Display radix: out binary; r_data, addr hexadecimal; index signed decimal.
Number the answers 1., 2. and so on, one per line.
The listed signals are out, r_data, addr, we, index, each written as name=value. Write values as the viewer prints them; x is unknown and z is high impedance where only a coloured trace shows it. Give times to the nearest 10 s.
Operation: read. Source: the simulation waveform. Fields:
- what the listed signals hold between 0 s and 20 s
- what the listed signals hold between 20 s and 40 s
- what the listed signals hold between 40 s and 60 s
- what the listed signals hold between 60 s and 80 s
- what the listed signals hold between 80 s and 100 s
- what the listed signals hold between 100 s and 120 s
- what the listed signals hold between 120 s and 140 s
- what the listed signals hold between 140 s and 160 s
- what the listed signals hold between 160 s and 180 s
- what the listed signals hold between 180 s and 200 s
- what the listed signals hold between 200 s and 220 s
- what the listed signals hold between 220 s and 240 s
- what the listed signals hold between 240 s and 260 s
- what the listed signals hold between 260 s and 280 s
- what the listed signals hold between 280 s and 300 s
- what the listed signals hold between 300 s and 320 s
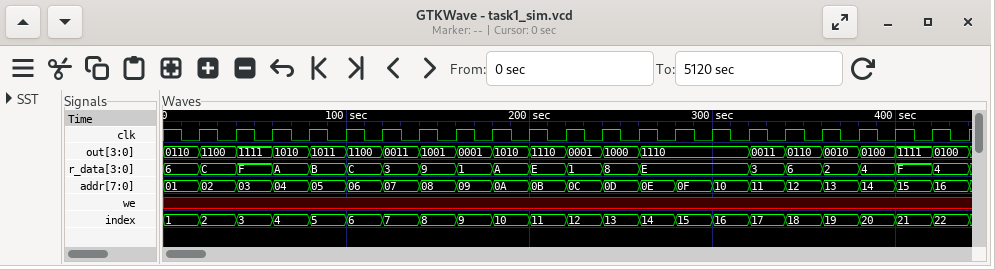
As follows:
1. out=0110, r_data=6, addr=01, we=x, index=1
2. out=1100, r_data=C, addr=02, we=x, index=2
3. out=1111, r_data=F, addr=03, we=x, index=3
4. out=1010, r_data=A, addr=04, we=x, index=4
5. out=1011, r_data=B, addr=05, we=x, index=5
6. out=1100, r_data=C, addr=06, we=x, index=6
7. out=0011, r_data=3, addr=07, we=x, index=7
8. out=1001, r_data=9, addr=08, we=x, index=8
9. out=0001, r_data=1, addr=09, we=x, index=9
10. out=1010, r_data=A, addr=0A, we=x, index=10
11. out=1110, r_data=E, addr=0B, we=x, index=11
12. out=0001, r_data=1, addr=0C, we=x, index=12
13. out=1000, r_data=8, addr=0D, we=x, index=13
14. out=1110, r_data=E, addr=0E, we=x, index=14
15. out=1110, r_data=E, addr=0F, we=x, index=15
16. out=1110, r_data=E, addr=10, we=x, index=16
